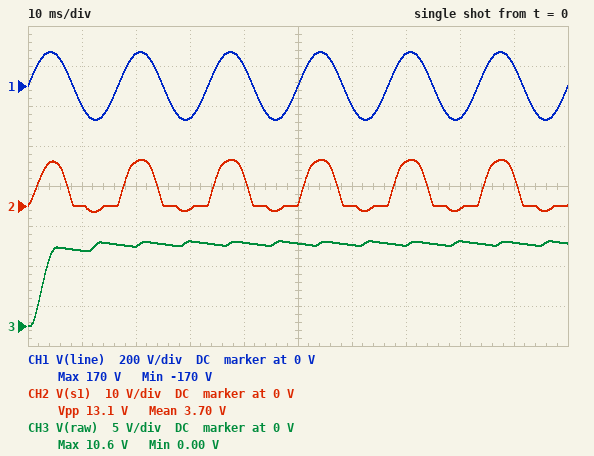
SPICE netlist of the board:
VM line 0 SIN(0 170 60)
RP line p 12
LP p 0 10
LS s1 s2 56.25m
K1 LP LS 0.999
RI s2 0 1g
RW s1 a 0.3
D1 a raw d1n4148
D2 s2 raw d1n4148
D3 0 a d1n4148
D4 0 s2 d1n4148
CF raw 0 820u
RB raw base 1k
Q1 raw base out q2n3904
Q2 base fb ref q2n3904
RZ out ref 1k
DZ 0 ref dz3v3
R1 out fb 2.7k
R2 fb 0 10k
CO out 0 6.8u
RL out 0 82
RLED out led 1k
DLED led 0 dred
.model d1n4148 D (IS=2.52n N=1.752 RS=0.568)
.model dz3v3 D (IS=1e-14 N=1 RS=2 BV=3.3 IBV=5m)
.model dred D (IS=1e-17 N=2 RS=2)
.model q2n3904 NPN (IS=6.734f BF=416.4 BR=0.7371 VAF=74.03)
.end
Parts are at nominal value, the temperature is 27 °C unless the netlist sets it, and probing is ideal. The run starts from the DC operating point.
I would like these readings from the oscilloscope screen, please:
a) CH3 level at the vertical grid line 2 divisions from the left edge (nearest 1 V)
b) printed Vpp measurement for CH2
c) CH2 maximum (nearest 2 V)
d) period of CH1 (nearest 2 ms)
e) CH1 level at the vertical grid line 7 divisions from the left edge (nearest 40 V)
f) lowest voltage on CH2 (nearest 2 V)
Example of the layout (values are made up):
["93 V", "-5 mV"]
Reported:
["10 V", "13.1 V", "12 V", "16 ms", "160 V", "-2 V"]
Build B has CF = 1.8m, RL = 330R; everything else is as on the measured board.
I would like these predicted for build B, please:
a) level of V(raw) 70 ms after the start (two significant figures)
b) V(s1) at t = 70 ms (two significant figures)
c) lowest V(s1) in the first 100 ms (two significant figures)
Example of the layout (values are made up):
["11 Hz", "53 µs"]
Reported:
["11 V", "11 V", "-2.2 V"]
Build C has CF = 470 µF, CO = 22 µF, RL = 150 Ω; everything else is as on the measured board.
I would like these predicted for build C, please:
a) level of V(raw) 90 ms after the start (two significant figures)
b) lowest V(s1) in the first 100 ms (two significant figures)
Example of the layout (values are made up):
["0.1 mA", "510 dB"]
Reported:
["11 V", "-1.2 V"]
